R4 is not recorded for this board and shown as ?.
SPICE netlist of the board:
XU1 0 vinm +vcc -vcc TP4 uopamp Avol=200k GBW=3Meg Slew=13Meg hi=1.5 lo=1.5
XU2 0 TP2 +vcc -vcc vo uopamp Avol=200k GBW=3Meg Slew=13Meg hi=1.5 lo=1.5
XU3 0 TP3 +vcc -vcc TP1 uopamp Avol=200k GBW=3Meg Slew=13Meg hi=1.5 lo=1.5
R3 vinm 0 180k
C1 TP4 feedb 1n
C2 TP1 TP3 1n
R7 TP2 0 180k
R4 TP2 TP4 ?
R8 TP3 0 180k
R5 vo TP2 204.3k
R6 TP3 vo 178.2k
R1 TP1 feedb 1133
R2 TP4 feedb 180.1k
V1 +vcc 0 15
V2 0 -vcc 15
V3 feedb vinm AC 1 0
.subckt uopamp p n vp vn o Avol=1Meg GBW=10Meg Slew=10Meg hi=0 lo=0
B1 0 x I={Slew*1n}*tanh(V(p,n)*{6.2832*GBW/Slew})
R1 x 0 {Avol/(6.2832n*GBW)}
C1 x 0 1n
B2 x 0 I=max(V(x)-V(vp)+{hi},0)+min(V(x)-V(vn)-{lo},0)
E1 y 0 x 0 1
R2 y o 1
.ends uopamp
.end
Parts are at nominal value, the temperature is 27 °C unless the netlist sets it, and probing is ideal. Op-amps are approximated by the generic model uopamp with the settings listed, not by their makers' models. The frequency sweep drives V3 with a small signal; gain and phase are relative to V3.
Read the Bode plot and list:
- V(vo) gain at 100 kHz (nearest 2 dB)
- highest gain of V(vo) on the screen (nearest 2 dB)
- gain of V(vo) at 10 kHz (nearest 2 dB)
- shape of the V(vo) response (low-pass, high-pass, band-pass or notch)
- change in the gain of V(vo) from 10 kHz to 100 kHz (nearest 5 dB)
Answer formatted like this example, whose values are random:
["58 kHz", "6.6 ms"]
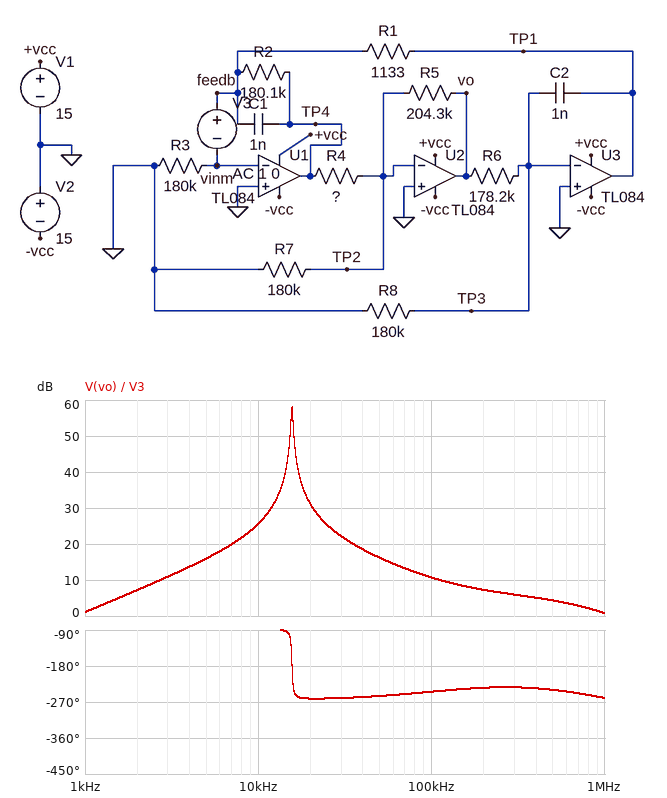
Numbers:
["10 dB", "58 dB", "26 dB", "band-pass", "-15 dB"]
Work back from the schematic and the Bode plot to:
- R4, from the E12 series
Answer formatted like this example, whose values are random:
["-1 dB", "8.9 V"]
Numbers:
["100 kΩ"]
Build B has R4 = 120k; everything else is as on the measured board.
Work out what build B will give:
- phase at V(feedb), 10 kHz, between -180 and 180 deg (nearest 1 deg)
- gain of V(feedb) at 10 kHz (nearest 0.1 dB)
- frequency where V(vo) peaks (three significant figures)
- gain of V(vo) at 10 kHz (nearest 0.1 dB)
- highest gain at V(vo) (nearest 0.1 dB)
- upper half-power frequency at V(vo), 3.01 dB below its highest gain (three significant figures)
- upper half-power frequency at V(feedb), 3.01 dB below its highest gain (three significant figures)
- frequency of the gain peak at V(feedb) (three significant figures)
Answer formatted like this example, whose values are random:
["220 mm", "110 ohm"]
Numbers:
["0 deg", "0.4 dB", "14.3 kHz", "26.9 dB", "54.2 dB", "14.5 kHz", "14.4 kHz", "14.2 kHz"]
